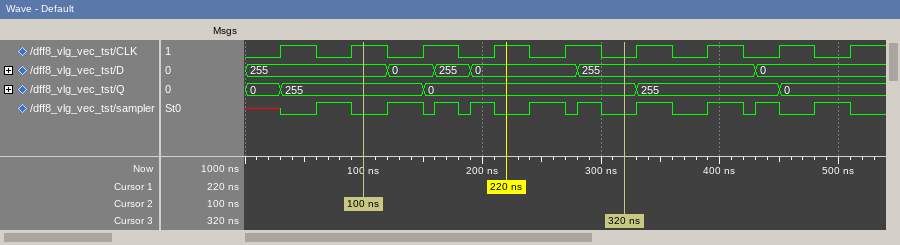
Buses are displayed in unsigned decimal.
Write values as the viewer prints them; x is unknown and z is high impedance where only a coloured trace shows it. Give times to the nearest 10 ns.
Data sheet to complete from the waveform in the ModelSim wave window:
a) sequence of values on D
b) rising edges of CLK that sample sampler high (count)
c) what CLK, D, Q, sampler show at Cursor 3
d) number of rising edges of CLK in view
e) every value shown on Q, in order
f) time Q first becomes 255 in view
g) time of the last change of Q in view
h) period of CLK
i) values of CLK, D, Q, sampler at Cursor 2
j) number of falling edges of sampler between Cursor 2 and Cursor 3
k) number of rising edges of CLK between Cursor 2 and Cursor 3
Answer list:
255, 0, 255, 0, 255, 0
6
CLK=0, D=255, Q=0, sampler=0
9
0, 255, 0, 255, 0
30 ns
450 ns
60 ns
CLK=1, D=255, Q=255, sampler=0
5
3
